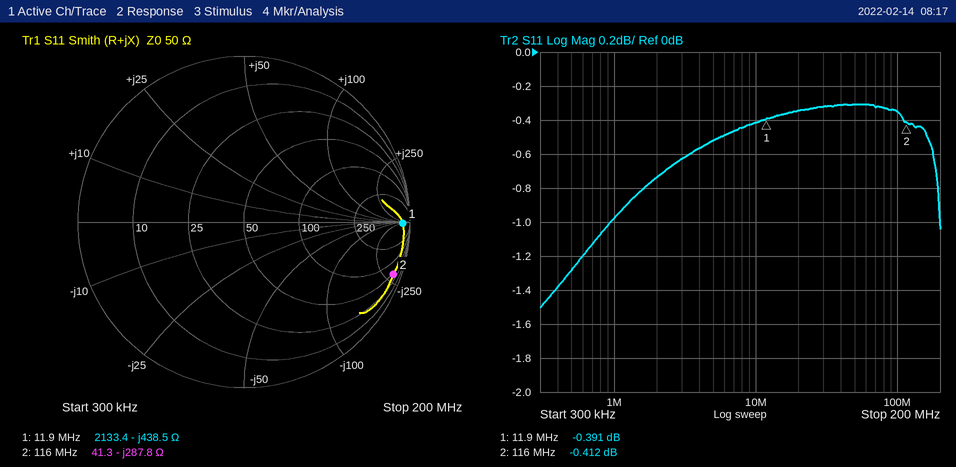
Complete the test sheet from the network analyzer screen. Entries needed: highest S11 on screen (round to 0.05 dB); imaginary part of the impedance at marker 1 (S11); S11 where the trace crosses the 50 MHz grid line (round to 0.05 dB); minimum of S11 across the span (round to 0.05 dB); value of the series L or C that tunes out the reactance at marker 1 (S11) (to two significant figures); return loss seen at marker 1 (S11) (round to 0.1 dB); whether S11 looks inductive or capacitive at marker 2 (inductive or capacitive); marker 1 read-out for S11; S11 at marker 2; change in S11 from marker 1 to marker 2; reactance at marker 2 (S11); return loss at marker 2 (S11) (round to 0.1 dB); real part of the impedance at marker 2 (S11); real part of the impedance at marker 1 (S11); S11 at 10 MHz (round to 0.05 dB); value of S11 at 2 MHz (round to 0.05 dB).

-0.30 dB
-438.5 Ω
-0.30 dB
-1.50 dB
5.9 µH
0.4 dB
capacitive
-0.391 dB
-0.412 dB
-0.021 dB
-287.8 Ω
0.4 dB
41.3 Ω
2133.4 Ω
-0.40 dB
-0.75 dB
